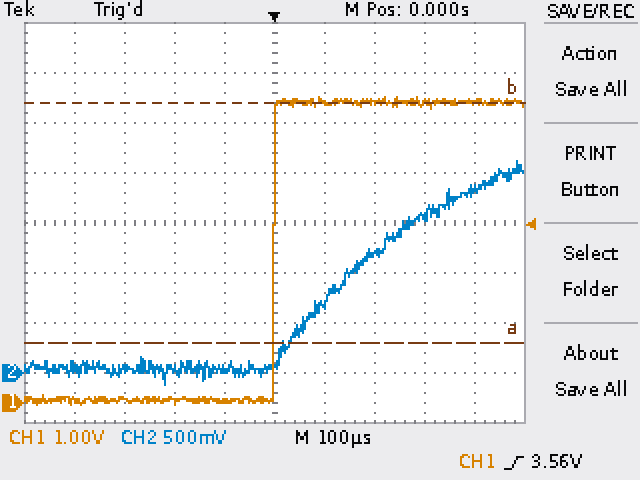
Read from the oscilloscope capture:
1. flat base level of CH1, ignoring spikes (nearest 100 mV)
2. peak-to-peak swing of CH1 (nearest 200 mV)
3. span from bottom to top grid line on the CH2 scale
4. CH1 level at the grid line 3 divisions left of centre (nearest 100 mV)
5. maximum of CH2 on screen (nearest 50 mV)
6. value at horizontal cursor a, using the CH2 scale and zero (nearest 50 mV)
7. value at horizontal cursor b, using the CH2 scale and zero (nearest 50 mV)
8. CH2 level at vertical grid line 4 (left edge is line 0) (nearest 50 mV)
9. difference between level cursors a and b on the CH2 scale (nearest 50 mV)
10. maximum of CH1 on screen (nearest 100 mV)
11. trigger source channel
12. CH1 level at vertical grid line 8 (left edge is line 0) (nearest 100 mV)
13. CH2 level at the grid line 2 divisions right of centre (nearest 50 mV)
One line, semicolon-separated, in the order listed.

100 mV; 6.2 V; 4 V; 100 mV; 2.10 V; 300 mV; 2.70 V; 50 mV; 2.40 V; 6.1 V; CH1; 6.0 V; 1.20 V
